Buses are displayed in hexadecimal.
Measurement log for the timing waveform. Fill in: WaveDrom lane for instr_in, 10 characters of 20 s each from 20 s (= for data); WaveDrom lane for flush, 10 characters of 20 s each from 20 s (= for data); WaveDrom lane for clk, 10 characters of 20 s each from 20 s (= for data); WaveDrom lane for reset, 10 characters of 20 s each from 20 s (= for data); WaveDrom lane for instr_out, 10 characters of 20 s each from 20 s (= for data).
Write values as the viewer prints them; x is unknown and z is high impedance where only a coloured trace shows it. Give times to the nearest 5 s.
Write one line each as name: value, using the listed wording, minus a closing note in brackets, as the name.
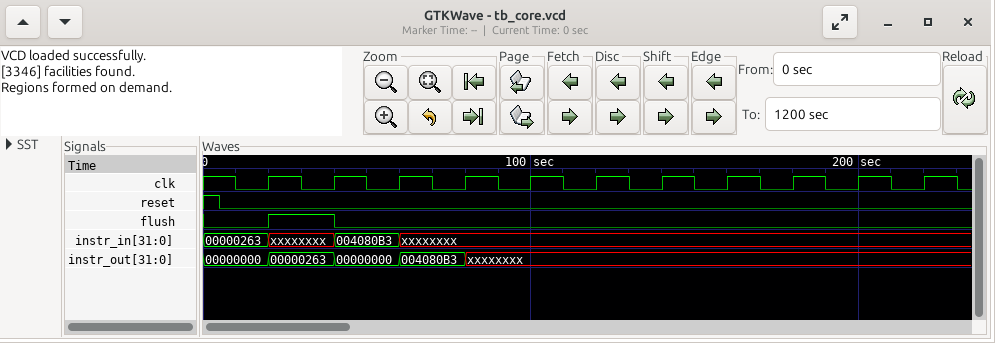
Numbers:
WaveDrom lane for instr_in, 10 characters of 20 s each from 20 s: {name: 'instr_in', wave: 'x=x.......', data: '004080B3'}
WaveDrom lane for flush, 10 characters of 20 s each from 20 s: {name: 'flush', wave: '10........'}
WaveDrom lane for clk, 10 characters of 20 s each from 20 s: {name: 'clk', wave: 'p.........'}
WaveDrom lane for reset, 10 characters of 20 s each from 20 s: {name: 'reset', wave: '0.........'}
WaveDrom lane for instr_out, 10 characters of 20 s each from 20 s: {name: 'instr_out', wave: '===x......', data: '00000263 00000000 004080B3'}
